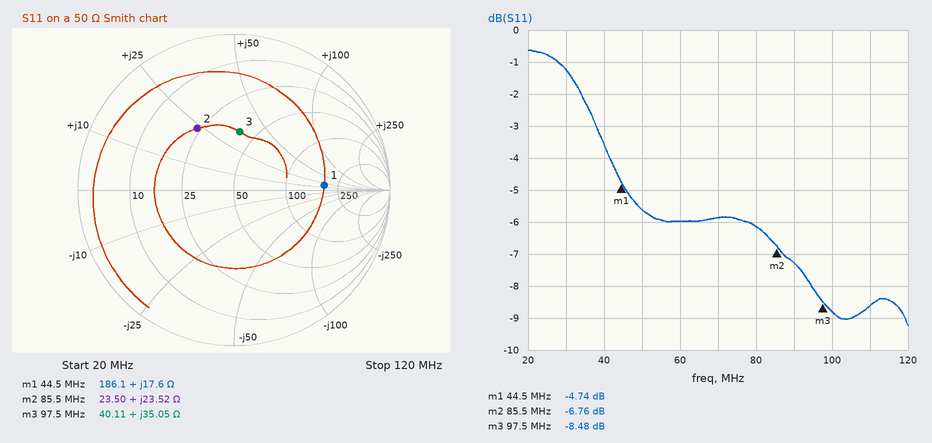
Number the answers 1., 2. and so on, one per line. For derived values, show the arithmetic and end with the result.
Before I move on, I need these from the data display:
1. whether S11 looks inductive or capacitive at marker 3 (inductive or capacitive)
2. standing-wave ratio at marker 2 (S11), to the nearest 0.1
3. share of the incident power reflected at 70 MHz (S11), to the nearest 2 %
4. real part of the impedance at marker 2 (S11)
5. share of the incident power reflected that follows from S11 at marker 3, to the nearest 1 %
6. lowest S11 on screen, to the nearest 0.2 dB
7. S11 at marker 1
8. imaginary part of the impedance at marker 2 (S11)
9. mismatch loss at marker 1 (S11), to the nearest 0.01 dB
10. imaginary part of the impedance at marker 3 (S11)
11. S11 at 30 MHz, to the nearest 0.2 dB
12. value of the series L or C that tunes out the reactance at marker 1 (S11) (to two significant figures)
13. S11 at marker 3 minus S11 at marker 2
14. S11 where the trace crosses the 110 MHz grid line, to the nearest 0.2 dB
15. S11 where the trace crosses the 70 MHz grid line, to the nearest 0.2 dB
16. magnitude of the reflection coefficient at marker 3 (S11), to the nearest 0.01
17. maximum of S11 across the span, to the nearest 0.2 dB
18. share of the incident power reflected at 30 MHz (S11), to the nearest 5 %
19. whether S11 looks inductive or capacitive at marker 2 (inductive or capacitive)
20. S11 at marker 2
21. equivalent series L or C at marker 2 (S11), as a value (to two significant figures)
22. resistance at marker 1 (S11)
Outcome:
1. inductive
2. 2.7
3. 10^(-5.8/10) ≈ 26 %
4. 23.50 Ω
5. 10^(-8.48/10) ≈ 14 %
6. -9.2 dB
7. -4.74 dB
8. +23.52 Ω
9. −10 log10(1 − 10^(-4.74/10)) ≈ 1.78 dB
10. +35.05 Ω
11. -1.2 dB
12. C = 1/(2π × 44.5 MHz × 17.6 Ω) ≈ 203 pF, so 200 pF to two significant figures
13. -8.48 − (-6.76) = -1.72 dB
14. -8.6 dB
15. -5.8 dB
16. 0.38
17. -0.6 dB
18. 10^(-1.2/10) ≈ 75.9 %, so 75 % to the nearest 5 %
19. inductive
20. -6.76 dB
21. L = 23.52 Ω/(2π × 85.5 MHz) ≈ 44 nH
22. 186.1 Ω
